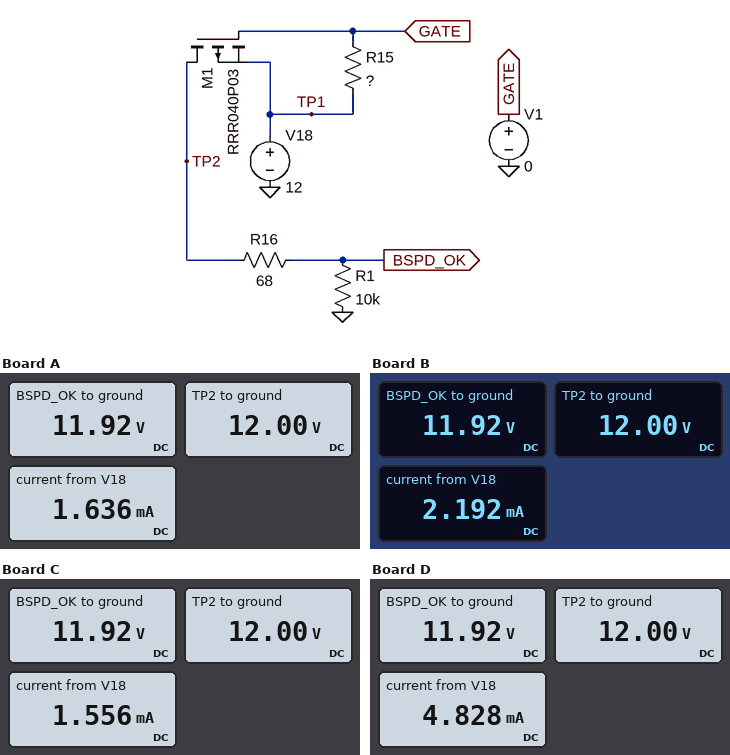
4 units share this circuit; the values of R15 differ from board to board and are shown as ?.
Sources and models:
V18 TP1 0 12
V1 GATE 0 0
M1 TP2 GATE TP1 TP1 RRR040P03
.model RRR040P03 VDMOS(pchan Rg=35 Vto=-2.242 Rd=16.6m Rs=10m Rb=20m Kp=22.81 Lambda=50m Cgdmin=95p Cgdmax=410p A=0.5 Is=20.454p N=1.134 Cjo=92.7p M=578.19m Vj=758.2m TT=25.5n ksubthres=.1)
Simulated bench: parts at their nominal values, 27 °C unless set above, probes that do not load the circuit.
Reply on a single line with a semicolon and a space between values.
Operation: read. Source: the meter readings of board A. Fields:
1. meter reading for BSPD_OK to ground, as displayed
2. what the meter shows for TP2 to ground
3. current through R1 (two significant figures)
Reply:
11.92 V; 12.00 V; 1.2 mA
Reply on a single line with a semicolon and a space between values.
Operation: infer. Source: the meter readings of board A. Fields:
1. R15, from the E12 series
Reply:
27 kΩ
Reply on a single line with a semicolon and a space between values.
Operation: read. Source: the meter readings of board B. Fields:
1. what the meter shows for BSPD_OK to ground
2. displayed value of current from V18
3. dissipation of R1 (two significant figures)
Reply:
11.92 V; 2.192 mA; 14 mW
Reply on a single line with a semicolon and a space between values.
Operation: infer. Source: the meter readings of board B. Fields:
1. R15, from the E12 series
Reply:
12 kΩ
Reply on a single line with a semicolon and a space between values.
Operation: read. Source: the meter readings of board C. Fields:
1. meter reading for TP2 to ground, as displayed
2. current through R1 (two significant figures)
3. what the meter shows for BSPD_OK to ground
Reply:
12.00 V; 1.2 mA; 11.92 V
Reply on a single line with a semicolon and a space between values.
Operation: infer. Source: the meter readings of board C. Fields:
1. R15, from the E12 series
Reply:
33 kΩ
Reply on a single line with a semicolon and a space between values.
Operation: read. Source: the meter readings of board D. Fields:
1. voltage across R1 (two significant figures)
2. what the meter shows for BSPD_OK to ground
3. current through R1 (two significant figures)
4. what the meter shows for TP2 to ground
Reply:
12 V; 11.92 V; 1.2 mA; 12.00 V
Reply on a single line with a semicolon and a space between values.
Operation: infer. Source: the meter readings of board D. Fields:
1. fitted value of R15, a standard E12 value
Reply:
3.3 kΩ
